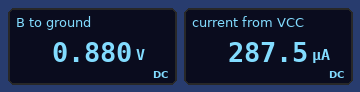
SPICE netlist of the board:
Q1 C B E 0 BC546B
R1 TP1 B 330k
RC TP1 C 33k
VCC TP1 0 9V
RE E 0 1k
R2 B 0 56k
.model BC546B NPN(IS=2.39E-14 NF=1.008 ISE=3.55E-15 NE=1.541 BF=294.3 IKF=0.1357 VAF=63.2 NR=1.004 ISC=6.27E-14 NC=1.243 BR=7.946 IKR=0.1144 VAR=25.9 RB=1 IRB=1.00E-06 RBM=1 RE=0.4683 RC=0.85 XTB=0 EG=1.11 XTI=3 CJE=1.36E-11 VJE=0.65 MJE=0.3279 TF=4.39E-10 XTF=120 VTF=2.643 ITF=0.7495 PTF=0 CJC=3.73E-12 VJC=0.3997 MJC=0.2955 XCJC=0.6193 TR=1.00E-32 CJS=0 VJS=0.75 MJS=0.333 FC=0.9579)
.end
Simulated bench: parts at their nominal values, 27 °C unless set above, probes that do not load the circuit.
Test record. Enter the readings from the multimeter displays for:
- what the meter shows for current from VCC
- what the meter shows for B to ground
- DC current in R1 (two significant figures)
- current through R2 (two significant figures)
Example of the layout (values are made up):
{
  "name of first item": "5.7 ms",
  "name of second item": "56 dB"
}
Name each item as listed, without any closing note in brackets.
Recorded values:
{
  "what the meter shows for current from VCC": "287.5 µA",
  "what the meter shows for B to ground": "0.880 V",
  "DC current in R1": "25 µA",
  "current through R2": "16 µA"
}
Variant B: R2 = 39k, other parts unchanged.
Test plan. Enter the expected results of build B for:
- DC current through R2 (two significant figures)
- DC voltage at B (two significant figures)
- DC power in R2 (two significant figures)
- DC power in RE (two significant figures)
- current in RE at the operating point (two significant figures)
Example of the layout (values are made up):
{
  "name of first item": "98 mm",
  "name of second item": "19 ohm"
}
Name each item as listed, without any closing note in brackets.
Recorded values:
{
  "DC current through R2": "22 µA",
  "DC voltage at B": "870 mV",
  "DC power in R2": "19 µW",
  "DC power in RE": "70 µW",
  "current in RE at the operating point": "260 µA"
}
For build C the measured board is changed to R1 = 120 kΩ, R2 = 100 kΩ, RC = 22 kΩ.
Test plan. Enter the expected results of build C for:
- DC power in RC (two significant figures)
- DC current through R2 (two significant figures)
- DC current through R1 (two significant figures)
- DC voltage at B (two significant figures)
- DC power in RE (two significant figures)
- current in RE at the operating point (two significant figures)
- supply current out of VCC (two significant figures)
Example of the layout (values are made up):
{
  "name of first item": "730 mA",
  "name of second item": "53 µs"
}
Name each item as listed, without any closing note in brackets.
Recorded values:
{
  "DC power in RC": "3.3 mW",
  "DC current through R2": "11 µA",
  "DC current through R1": "66 µA",
  "DC voltage at B": "1.1 V",
  "DC power in RE": "200 µW",
  "current in RE at the operating point": "440 µA",
  "supply current out of VCC": "450 µA"
}
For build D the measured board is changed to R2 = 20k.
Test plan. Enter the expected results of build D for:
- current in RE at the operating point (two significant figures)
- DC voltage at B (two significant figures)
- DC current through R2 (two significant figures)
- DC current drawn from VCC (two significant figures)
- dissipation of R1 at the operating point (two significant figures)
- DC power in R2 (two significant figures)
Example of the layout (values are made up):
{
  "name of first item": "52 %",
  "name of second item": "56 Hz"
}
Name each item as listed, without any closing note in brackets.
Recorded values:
{
  "current in RE at the operating point": "7.3 µA",
  "DC voltage at B": "510 mV",
  "DC current through R2": "26 µA",
  "DC current drawn from VCC": "33 µA",
  "dissipation of R1 at the operating point": "220 µW",
  "DC power in R2": "13 µW"
}
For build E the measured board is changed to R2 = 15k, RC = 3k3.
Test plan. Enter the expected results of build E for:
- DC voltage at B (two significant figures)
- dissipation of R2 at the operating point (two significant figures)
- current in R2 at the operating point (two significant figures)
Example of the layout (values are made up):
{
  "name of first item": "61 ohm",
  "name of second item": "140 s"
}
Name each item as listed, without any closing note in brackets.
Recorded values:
{
  "DC voltage at B": "390 mV",
  "dissipation of R2 at the operating point": "10 µW",
  "current in R2 at the operating point": "26 µA"
}
